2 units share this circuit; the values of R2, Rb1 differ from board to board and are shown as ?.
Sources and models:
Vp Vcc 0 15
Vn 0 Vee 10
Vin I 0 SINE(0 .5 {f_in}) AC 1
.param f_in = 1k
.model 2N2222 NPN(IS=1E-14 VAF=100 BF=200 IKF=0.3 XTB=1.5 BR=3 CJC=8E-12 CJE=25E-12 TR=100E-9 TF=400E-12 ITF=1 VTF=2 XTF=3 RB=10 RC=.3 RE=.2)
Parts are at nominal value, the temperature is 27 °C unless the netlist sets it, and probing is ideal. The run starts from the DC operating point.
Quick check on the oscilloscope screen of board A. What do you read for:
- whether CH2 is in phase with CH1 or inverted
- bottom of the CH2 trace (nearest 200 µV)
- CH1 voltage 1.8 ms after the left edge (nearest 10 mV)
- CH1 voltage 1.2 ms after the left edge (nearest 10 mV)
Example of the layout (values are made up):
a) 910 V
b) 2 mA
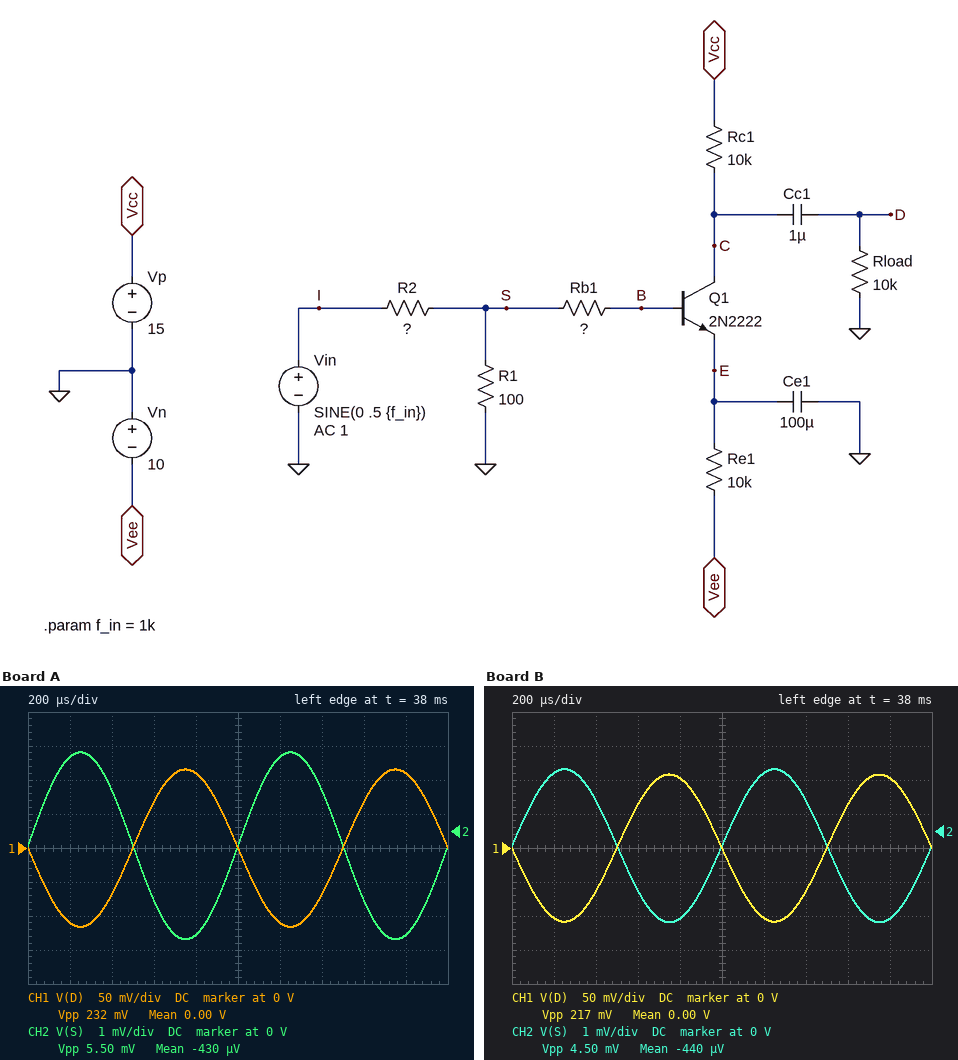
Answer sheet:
a) inverted
b) -3.2 mV
c) 110 mV
d) -110 mV
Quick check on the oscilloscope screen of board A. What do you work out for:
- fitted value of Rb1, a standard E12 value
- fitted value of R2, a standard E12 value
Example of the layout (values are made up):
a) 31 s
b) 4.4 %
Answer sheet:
a) 18 kΩ
b) 18 kΩ
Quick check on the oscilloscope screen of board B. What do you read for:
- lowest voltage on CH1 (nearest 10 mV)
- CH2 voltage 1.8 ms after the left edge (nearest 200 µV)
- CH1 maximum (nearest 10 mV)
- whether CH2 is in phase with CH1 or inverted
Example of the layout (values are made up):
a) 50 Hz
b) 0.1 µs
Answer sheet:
a) -110 mV
b) -2.6 mV
c) 110 mV
d) inverted
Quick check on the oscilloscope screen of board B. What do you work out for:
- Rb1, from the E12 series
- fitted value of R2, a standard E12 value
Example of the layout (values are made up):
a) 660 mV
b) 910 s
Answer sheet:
a) 15 kΩ
b) 22 kΩ
